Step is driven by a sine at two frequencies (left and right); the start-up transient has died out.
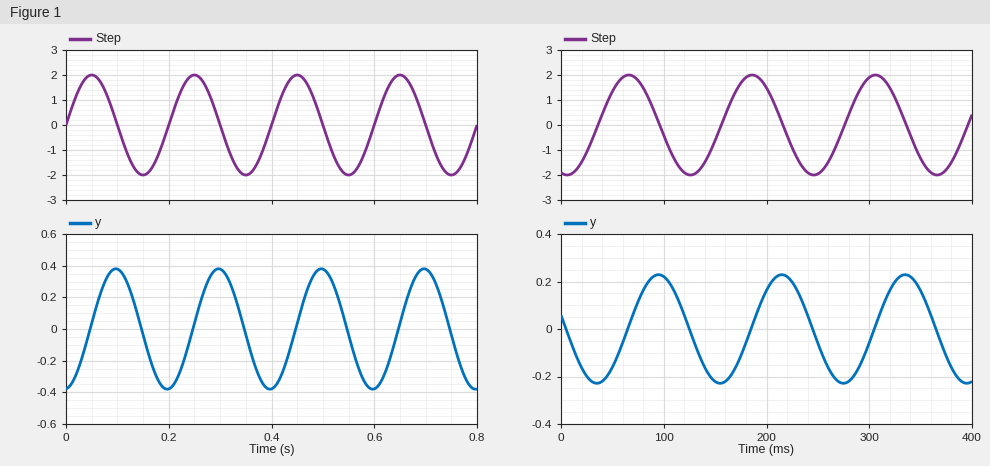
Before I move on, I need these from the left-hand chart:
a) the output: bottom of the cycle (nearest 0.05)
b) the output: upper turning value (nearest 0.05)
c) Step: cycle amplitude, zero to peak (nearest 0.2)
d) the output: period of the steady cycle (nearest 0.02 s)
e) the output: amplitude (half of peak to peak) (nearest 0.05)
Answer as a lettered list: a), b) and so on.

a) -0.40
b) 0.40
c) 2.0
d) 0.20 s
e) 0.40
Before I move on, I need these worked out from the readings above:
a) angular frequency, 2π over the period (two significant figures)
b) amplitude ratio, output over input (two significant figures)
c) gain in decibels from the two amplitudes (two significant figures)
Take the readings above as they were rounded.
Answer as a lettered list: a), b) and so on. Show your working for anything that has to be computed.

a) 2π / 0.2 = 31 rad/s
b) 0.4 / 2 = 0.20
c) 20 log10(0.4 / 2) = -14 dB
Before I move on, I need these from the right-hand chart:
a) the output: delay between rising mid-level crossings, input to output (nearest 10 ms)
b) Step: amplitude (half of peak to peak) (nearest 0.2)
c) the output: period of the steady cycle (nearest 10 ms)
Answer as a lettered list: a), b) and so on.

a) 30 ms
b) 2.0
c) 120 ms
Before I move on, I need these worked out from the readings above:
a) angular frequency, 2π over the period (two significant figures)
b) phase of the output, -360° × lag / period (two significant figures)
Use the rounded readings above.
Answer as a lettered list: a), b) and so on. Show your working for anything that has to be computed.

a) 2π / 120 = 0.052 rad/ms
b) -360 × 30 / 120 = -90°
